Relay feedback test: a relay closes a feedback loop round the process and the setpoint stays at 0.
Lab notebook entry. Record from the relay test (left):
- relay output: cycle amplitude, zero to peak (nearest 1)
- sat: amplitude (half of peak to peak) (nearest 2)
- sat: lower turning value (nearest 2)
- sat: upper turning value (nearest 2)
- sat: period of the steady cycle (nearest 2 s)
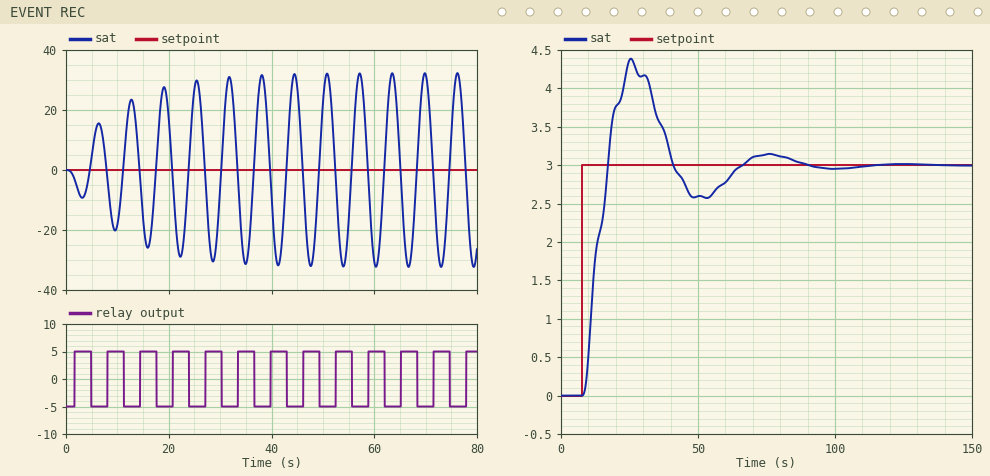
5
32
-32
32
6 s
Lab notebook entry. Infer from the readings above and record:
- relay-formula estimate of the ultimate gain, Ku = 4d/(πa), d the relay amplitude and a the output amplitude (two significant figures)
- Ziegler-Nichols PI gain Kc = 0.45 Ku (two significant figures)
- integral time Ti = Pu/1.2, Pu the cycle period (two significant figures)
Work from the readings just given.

0.20
0.090
5.0 s
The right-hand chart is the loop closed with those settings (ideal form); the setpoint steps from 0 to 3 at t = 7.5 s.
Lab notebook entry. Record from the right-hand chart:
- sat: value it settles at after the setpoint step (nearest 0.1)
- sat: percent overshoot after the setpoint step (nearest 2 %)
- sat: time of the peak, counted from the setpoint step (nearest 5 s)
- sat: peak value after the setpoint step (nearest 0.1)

3.0
46 %
20 s
4.4
